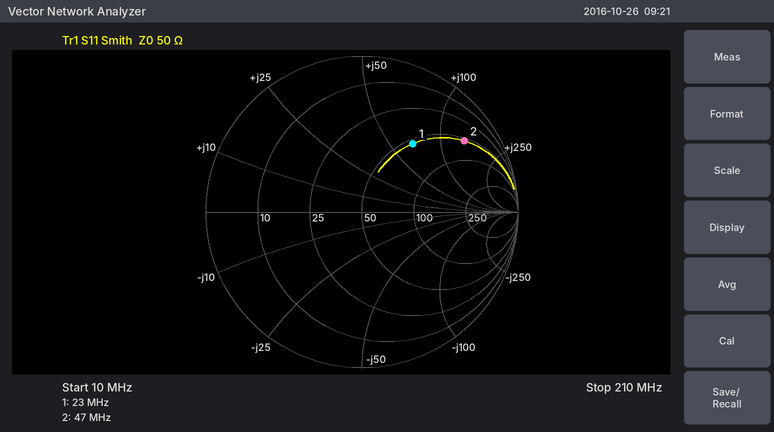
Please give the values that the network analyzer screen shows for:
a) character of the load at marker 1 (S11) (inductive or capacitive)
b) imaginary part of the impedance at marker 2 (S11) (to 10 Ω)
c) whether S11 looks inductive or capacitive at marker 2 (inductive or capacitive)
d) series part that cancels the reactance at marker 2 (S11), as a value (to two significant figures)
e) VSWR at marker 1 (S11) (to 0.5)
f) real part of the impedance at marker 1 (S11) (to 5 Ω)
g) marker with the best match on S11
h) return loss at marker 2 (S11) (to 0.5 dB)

inductive
+140 Ω
inductive
24 pF
3.5
55 Ω
marker 1
2.0 dB
